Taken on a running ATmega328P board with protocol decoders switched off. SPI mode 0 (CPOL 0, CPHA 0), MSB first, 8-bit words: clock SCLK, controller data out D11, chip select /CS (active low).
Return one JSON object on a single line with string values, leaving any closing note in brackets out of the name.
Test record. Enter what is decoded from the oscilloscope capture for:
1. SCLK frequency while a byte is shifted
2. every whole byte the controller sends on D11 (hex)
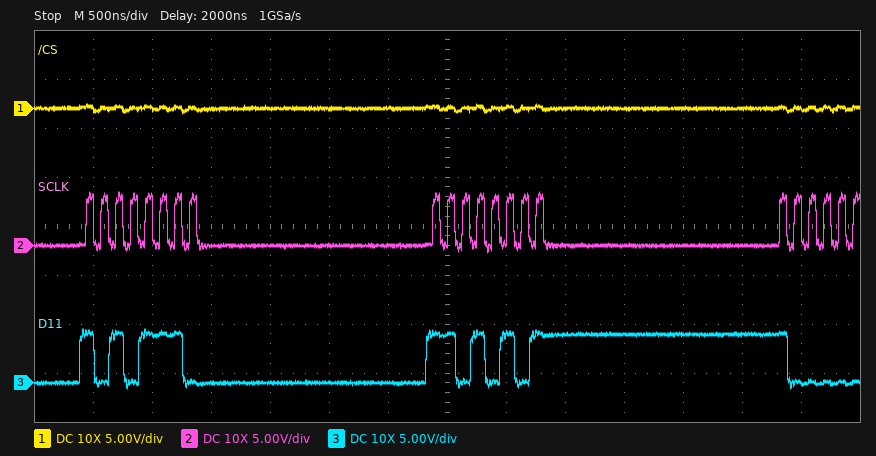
{"SCLK frequency while a byte is shifted": "8 MHz", "every whole byte the controller sends on D11": "0xAE 0xD5"}
